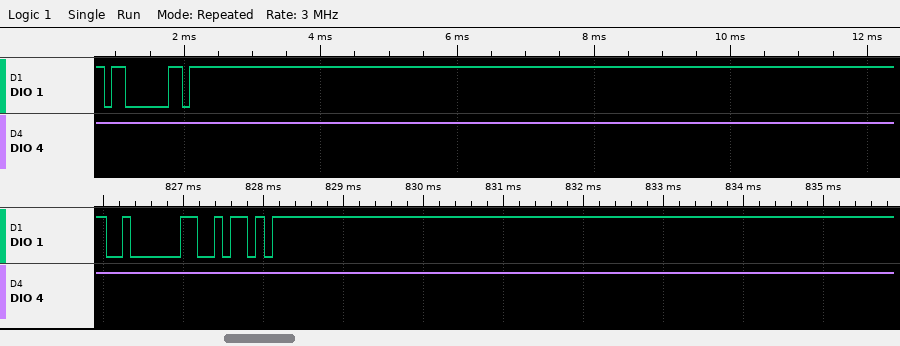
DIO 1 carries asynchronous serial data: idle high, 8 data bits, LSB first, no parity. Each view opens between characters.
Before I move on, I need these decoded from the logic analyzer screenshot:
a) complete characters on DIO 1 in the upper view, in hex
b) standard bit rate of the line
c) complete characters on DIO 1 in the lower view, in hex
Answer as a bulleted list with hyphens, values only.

- 03, FF
- 9600 baud
- 02, 5A
